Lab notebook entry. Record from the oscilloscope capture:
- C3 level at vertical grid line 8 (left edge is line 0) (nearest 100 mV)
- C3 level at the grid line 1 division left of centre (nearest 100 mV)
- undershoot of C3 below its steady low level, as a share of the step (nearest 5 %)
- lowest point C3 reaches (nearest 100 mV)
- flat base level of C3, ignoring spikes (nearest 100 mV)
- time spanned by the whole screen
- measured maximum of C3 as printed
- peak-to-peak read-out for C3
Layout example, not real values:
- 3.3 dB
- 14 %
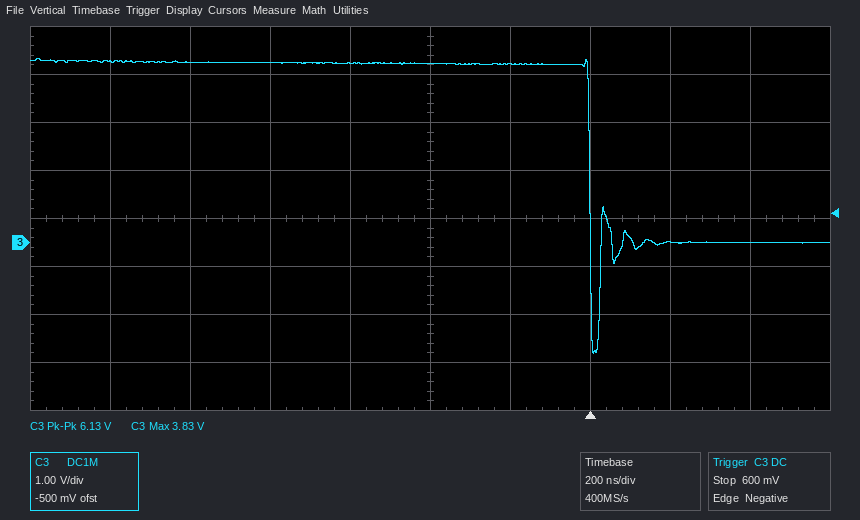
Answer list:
- 0.0 V
- 3.7 V
- 60 %
- -2.3 V
- 0.0 V
- 2 µs
- 3.83 V
- 6.13 V
